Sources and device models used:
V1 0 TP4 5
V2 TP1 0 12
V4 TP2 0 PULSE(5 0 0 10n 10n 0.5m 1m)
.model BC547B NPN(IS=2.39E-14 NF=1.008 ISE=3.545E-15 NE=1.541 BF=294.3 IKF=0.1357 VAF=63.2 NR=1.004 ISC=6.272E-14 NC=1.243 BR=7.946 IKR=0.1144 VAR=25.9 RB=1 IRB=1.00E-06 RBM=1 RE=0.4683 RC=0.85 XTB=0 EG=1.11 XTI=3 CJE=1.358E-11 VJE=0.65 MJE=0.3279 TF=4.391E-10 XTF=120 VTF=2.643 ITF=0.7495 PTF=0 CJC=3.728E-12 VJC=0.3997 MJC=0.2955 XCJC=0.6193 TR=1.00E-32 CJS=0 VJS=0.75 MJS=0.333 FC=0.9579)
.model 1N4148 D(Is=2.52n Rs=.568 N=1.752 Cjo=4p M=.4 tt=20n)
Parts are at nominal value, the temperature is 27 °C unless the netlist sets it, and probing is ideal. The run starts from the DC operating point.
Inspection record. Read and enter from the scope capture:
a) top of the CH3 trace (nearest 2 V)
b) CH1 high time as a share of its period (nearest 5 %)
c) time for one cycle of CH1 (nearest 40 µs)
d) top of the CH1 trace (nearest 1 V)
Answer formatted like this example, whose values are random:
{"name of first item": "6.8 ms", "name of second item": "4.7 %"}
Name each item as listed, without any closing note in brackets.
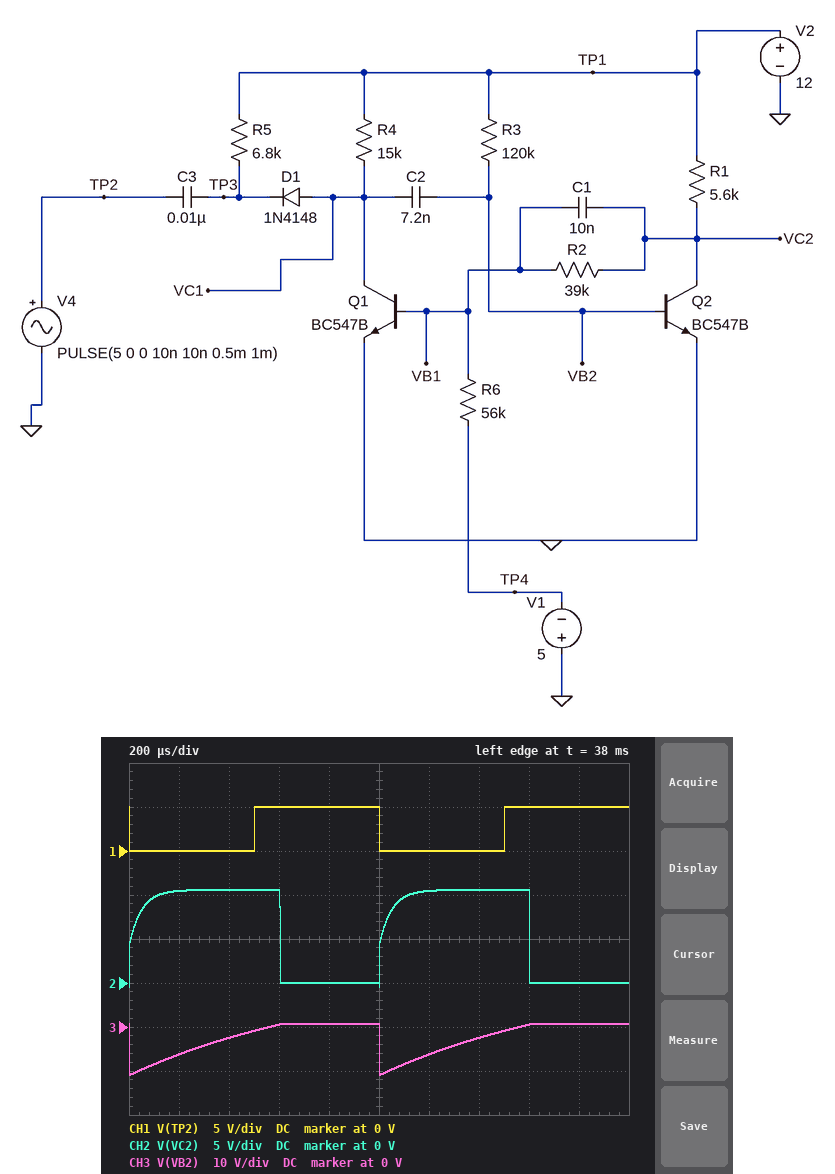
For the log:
{"top of the CH3 trace": "0 V", "CH1 high time as a share of its period": "50 %", "time for one cycle of CH1": "1.00 ms", "top of the CH1 trace": "5 V"}
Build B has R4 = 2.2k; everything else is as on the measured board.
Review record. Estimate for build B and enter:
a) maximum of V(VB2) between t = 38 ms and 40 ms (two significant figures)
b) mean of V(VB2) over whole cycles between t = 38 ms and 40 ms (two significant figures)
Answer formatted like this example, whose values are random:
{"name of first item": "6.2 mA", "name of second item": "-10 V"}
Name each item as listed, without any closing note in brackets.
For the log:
{"maximum of V(VB2) between t = 38 ms and 40 ms": "750 mV", "mean of V(VB2) over whole cycles between t = 38 ms and 40 ms": "-2.6 V"}
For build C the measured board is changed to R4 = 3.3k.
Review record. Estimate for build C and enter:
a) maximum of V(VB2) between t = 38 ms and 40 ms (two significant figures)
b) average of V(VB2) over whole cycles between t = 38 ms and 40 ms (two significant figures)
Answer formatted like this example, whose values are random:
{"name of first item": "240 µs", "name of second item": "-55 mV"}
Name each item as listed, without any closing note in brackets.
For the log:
{"maximum of V(VB2) between t = 38 ms and 40 ms": "740 mV", "average of V(VB2) over whole cycles between t = 38 ms and 40 ms": "-2.6 V"}
